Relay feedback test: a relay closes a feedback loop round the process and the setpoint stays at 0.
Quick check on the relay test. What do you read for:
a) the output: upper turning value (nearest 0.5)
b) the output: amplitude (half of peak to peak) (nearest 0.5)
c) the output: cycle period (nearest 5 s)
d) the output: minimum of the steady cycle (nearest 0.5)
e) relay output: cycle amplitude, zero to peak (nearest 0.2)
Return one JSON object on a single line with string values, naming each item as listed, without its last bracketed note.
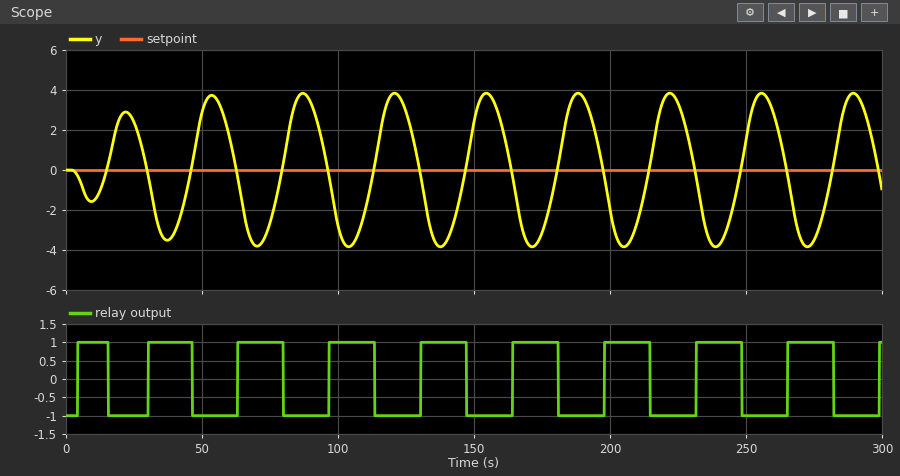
{"the output: upper turning value": "4.0", "the output: amplitude (half of peak to peak)": "4.0", "the output: cycle period": "35 s", "the output: minimum of the steady cycle": "-4.0", "relay output: cycle amplitude, zero to peak": "1.0"}
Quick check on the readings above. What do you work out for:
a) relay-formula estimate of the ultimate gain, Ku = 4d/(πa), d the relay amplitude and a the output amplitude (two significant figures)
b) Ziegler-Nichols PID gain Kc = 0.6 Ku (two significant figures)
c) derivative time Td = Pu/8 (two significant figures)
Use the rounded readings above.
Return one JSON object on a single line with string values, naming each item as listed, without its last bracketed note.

{"relay-formula estimate of the ultimate gain, Ku = 4d/(πa), d the relay amplitude and a the output amplitude": "0.32", "Ziegler-Nichols PID gain Kc = 0.6 Ku": "0.19", "derivative time Td = Pu/8": "4.4 s"}
